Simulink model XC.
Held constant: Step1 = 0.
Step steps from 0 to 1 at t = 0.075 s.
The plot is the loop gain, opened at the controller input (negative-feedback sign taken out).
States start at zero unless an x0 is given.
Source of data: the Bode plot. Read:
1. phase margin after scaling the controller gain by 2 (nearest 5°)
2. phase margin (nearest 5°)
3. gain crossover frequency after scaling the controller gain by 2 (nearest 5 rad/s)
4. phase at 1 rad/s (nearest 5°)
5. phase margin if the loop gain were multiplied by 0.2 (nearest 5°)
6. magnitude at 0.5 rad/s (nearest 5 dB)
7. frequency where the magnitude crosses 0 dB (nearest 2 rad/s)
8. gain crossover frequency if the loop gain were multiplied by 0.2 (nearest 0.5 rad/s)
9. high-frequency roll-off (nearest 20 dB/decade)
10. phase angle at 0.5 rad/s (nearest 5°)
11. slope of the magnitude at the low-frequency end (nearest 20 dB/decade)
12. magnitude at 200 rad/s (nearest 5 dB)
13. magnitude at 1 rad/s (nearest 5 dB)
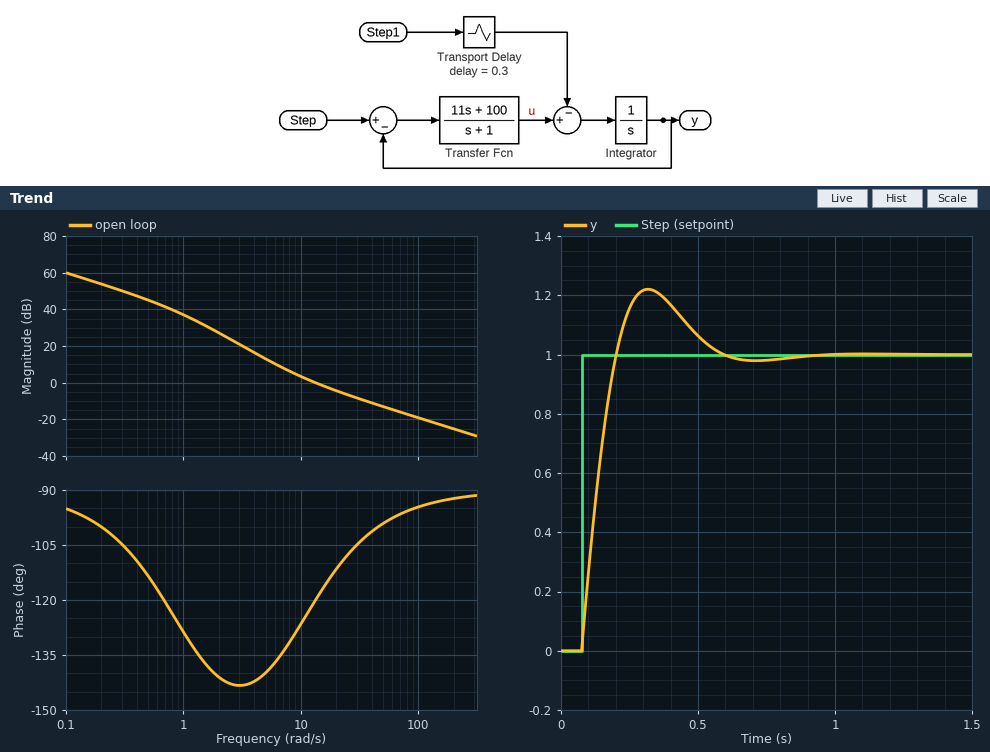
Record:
70°
60°
25 rad/s
-130°
40°
45 dB
14 rad/s
4.5 rad/s
-20 dB/decade
-115°
-20 dB/decade
-25 dB
35 dB
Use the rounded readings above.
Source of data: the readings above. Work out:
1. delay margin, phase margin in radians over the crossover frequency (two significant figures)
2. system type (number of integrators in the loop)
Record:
0.075 s
1
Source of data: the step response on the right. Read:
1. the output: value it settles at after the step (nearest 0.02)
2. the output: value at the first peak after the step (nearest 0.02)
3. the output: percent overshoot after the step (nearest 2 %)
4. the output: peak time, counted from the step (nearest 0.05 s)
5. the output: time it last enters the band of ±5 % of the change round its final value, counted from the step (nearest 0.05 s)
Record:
1.00
1.22
22 %
0.25 s
0.45 s
